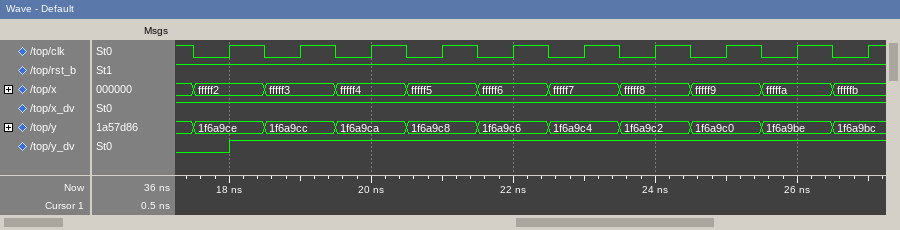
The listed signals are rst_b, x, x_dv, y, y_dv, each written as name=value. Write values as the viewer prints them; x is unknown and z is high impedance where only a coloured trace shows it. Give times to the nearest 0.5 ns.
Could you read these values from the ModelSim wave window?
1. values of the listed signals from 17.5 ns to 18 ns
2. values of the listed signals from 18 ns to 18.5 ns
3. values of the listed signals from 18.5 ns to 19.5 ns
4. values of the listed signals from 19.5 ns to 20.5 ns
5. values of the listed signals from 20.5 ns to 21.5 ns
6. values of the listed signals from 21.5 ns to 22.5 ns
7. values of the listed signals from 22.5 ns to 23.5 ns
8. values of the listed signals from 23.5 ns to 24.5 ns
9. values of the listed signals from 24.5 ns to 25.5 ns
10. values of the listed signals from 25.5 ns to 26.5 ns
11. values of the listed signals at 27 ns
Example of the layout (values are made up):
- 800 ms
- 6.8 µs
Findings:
- rst_b=1, x=fffff2, x_dv=1, y=1f6a9ce, y_dv=0
- rst_b=1, x=fffff2, x_dv=1, y=1f6a9ce, y_dv=1
- rst_b=1, x=fffff3, x_dv=1, y=1f6a9cc, y_dv=1
- rst_b=1, x=fffff4, x_dv=1, y=1f6a9ca, y_dv=1
- rst_b=1, x=fffff5, x_dv=1, y=1f6a9c8, y_dv=1
- rst_b=1, x=fffff6, x_dv=1, y=1f6a9c6, y_dv=1
- rst_b=1, x=fffff7, x_dv=1, y=1f6a9c4, y_dv=1
- rst_b=1, x=fffff8, x_dv=1, y=1f6a9c2, y_dv=1
- rst_b=1, x=fffff9, x_dv=1, y=1f6a9c0, y_dv=1
- rst_b=1, x=fffffa, x_dv=1, y=1f6a9be, y_dv=1
- rst_b=1, x=fffffb, x_dv=1, y=1f6a9bc, y_dv=1
